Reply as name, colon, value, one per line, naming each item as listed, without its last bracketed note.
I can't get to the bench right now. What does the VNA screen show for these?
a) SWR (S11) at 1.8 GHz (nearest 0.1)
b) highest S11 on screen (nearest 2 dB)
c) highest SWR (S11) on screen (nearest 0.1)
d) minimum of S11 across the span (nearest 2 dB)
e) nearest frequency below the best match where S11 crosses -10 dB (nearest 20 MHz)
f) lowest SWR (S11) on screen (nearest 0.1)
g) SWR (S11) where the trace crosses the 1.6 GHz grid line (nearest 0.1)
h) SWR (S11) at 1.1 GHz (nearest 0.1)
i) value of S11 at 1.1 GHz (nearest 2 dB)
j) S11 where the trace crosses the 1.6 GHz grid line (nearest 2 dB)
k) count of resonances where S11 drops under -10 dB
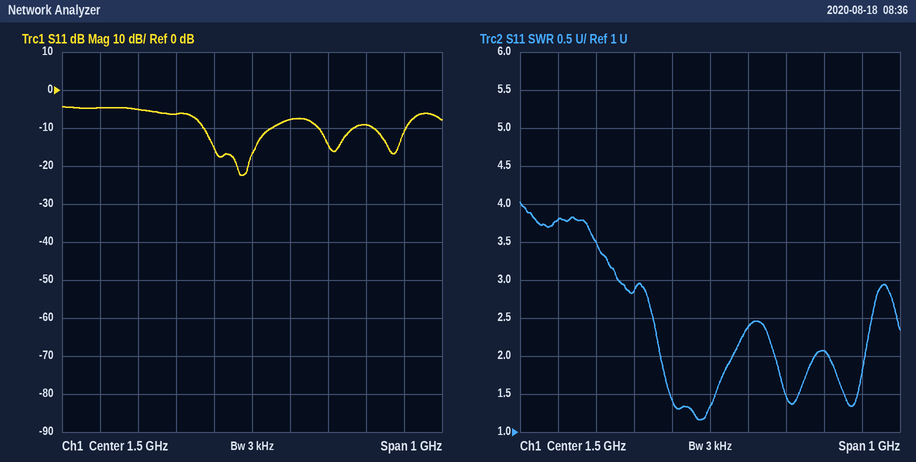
SWR (S11) at 1.8 GHz: 2.1
highest S11 on screen: -4 dB
highest SWR (S11) on screen: 4.0
minimum of S11 across the span: -22 dB
nearest frequency below the best match where S11 crosses -10 dB: 1.38 GHz
lowest SWR (S11) on screen: 1.2
SWR (S11) where the trace crosses the 1.6 GHz grid line: 2.4
SWR (S11) at 1.1 GHz: 3.8
value of S11 at 1.1 GHz: -4 dB
S11 where the trace crosses the 1.6 GHz grid line: -8 dB
count of resonances where S11 drops under -10 dB: 3
